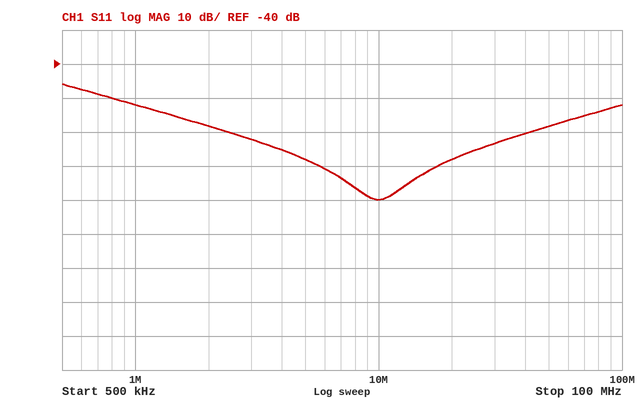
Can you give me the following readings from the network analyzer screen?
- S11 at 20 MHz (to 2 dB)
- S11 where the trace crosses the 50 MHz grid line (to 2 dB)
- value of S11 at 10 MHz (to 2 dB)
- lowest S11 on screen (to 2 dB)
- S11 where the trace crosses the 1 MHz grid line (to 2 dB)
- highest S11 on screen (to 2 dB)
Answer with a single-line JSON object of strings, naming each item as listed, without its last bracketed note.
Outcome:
{"S11 at 20 MHz": "-68 dB", "S11 where the trace crosses the 50 MHz grid line": "-58 dB", "value of S11 at 10 MHz": "-80 dB", "lowest S11 on screen": "-80 dB", "S11 where the trace crosses the 1 MHz grid line": "-52 dB", "highest S11 on screen": "-46 dB"}
